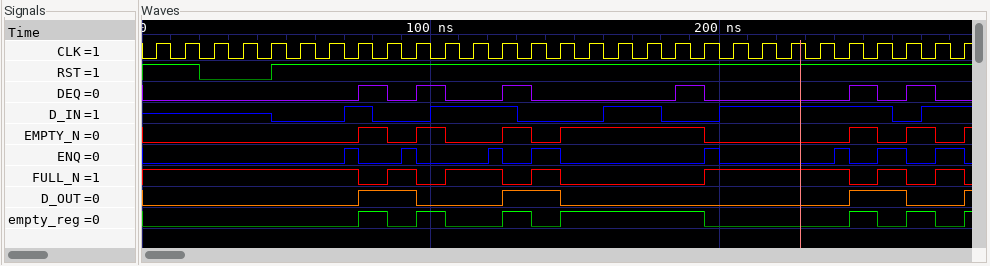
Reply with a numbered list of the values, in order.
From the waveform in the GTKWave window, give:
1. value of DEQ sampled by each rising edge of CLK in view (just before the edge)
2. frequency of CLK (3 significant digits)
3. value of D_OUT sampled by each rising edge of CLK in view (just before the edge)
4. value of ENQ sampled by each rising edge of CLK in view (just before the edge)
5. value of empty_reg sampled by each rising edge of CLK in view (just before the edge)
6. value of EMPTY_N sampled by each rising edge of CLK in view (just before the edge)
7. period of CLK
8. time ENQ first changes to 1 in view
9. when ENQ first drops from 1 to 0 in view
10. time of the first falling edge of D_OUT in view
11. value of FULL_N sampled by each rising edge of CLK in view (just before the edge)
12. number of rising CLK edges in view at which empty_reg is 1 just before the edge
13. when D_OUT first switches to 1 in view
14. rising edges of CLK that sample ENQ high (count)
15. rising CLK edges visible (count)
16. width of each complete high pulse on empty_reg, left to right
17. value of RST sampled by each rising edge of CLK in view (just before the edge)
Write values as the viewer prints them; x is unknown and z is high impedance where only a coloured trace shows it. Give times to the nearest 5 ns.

1. 0 0 0 0 0 0 0 0 1 0 1 0 0 1 0 0 0 0 0 1 0 0 0 0 0 1 0 1 0
2. 100 MHz
3. 0 0 0 0 0 0 0 0 1 1 0 0 0 1 1 0 0 0 0 0 0 0 0 0 0 1 1 0 0
4. 0 0 0 0 0 0 0 1 0 1 0 0 1 0 1 0 0 0 0 0 0 0 0 0 1 0 1 0 1
5. 0 0 0 0 0 0 0 0 1 0 1 0 0 1 0 1 1 1 1 1 0 0 0 0 0 1 0 1 0
6. 0 0 0 0 0 0 0 0 1 0 1 0 0 1 0 1 1 1 1 1 0 0 0 0 0 1 0 1 0
7. 10 ns
8. 70 ns
9. 75 ns
10. 95 ns
11. 1 1 1 1 1 1 1 1 0 1 0 1 1 0 1 0 0 0 0 0 1 1 1 1 1 0 1 0 1
12. 10
13. 75 ns
14. 7
15. 29
16. 10 ns, 10 ns, 10 ns, 50 ns, 10 ns, 10 ns
17. 1 1 0 0 0 1 1 1 1 1 1 1 1 1 1 1 1 1 1 1 1 1 1 1 1 1 1 1 1
